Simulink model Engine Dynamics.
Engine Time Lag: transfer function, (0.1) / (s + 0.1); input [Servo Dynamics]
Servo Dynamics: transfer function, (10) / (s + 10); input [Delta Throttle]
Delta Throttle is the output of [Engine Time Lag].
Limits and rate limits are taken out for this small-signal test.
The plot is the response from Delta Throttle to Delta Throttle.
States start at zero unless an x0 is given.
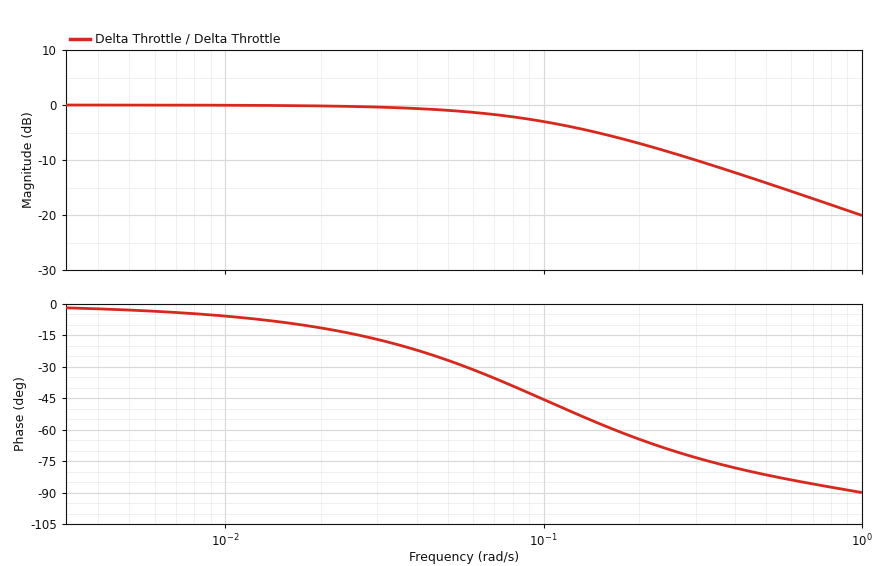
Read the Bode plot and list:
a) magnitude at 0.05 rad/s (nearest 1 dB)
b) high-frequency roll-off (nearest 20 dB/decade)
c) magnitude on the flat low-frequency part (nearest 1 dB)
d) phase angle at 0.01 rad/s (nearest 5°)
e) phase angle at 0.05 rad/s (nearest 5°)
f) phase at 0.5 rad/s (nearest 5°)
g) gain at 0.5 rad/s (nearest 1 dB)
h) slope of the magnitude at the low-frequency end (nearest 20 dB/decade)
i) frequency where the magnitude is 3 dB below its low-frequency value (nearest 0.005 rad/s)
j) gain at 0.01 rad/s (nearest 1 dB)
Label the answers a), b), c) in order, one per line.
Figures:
a) -1 dB
b) -20 dB/decade
c) 0 dB
d) -5°
e) -25°
f) -80°
g) -14 dB
h) 0 dB/decade
i) 0.100 rad/s
j) 0 dB
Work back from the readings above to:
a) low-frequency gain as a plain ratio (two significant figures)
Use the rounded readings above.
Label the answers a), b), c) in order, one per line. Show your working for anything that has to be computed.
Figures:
a) 10^(0 / 20) = 1.0
